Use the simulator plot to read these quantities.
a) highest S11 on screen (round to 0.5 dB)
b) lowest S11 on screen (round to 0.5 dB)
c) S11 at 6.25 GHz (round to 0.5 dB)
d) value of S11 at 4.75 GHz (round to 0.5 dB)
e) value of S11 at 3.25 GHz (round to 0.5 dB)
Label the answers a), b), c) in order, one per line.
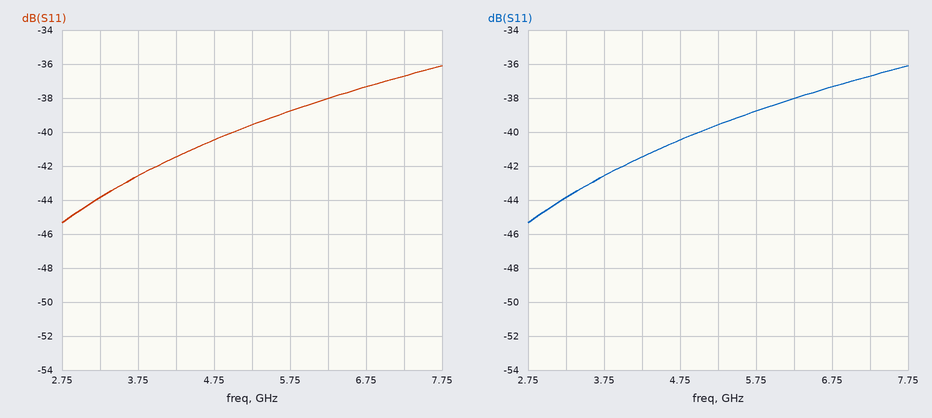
a) -36.0 dB
b) -45.5 dB
c) -38.0 dB
d) -40.5 dB
e) -44.0 dB
